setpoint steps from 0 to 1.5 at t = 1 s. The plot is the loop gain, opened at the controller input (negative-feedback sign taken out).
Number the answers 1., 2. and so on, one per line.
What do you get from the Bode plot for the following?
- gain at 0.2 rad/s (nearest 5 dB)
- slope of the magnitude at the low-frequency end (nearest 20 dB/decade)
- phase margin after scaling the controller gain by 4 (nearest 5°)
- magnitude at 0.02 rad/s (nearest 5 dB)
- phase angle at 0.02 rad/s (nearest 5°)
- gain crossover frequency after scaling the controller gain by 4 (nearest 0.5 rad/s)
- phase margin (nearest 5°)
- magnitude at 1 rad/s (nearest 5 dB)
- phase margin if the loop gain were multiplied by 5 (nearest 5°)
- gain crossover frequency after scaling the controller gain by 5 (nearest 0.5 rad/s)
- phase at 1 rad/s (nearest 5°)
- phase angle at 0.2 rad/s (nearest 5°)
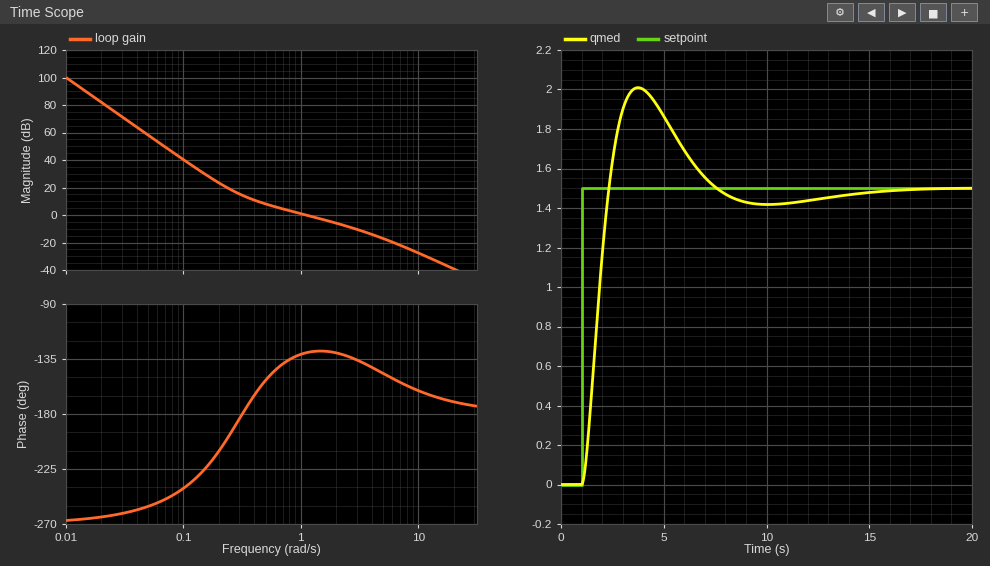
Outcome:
1. 25 dB
2. -60 dB/decade
3. 40°
4. 80 dB
5. -265°
6. 3.5 rad/s
7. 50°
8. 0 dB
9. 40°
10. 4.0 rad/s
11. -130°
12. -210°
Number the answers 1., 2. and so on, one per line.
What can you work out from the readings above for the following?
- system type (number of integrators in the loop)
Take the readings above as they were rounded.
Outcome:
1. 3
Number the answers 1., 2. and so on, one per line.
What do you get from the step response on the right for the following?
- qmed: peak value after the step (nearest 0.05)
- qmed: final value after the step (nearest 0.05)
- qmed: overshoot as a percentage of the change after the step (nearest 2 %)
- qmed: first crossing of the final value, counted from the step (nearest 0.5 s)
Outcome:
1. 2.00
2. 1.50
3. 34 %
4. 1.5 s
